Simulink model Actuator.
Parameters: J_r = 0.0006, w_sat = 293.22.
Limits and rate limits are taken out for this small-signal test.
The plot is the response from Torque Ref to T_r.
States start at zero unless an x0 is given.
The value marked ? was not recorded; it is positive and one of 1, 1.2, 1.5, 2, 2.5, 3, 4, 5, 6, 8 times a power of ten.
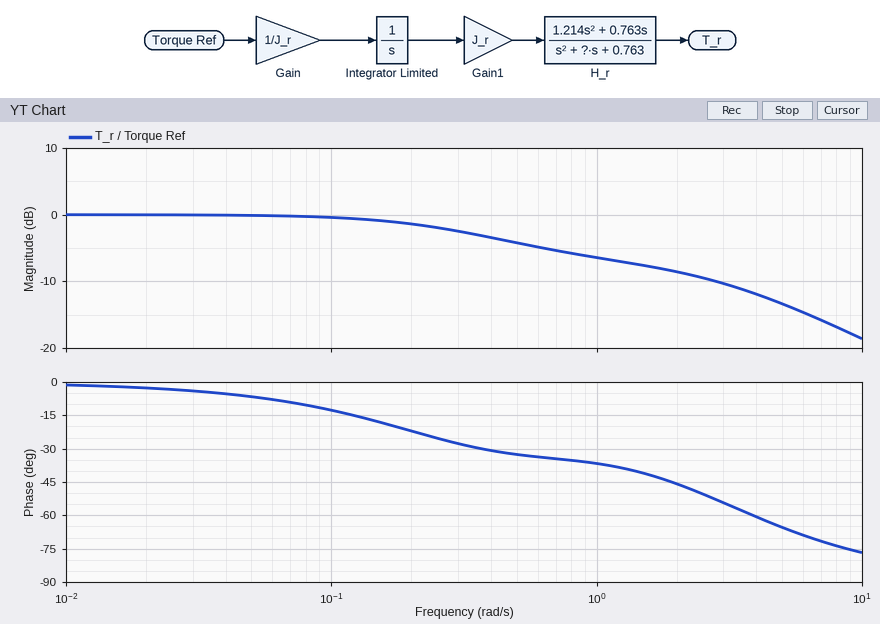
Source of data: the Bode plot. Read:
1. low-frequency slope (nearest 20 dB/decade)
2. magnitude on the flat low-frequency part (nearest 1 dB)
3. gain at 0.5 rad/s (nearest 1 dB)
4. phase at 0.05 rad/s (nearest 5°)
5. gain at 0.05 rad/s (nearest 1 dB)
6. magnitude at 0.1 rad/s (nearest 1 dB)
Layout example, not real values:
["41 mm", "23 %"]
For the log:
["0 dB/decade", "0 dB", "-4 dB", "-5°", "0 dB", "0 dB"]
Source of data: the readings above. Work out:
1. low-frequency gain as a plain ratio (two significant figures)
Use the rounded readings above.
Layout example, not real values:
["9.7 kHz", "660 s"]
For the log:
["1.0"]
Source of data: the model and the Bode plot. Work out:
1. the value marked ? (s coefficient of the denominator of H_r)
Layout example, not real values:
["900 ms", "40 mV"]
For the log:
["3"]
